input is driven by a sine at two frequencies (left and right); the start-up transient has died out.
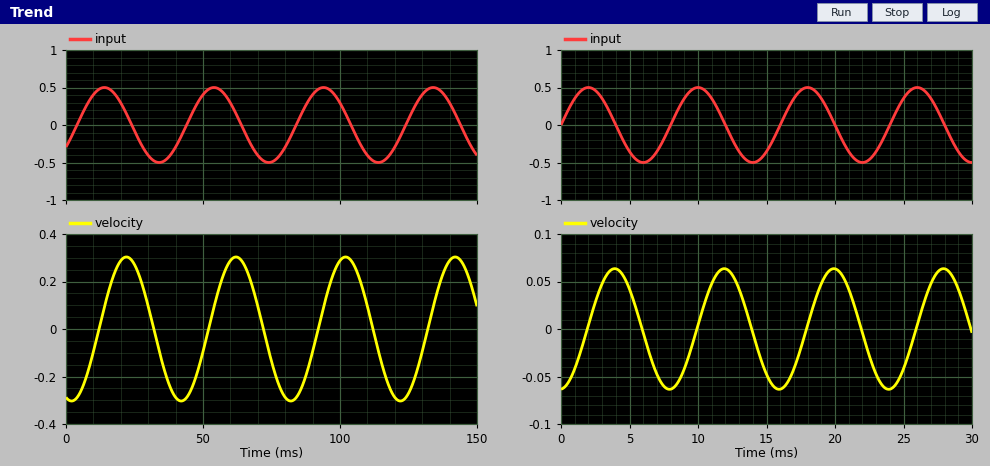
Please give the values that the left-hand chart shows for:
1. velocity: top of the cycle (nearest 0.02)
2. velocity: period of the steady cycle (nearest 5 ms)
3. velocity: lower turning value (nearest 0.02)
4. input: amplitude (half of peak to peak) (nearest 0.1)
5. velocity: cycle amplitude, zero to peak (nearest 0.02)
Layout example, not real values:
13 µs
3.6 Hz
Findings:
0.30
40 ms
-0.30
0.5
0.30
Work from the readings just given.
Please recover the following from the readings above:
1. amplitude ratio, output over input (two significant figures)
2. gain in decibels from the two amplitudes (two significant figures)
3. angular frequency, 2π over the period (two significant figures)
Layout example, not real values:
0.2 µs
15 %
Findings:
0.60
-4.4 dB
0.16 rad/ms
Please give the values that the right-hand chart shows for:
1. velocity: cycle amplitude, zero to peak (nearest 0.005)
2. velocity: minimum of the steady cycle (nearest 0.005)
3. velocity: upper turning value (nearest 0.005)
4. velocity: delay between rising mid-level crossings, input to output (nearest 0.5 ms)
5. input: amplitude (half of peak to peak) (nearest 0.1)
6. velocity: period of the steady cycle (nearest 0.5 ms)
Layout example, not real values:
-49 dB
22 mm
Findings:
0.065
-0.065
0.065
2.0 ms
0.5
8.0 ms
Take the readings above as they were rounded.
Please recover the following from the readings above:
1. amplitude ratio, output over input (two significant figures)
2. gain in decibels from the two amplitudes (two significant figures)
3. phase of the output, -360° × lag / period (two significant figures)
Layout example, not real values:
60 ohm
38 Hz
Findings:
0.13
-18 dB
-90°
